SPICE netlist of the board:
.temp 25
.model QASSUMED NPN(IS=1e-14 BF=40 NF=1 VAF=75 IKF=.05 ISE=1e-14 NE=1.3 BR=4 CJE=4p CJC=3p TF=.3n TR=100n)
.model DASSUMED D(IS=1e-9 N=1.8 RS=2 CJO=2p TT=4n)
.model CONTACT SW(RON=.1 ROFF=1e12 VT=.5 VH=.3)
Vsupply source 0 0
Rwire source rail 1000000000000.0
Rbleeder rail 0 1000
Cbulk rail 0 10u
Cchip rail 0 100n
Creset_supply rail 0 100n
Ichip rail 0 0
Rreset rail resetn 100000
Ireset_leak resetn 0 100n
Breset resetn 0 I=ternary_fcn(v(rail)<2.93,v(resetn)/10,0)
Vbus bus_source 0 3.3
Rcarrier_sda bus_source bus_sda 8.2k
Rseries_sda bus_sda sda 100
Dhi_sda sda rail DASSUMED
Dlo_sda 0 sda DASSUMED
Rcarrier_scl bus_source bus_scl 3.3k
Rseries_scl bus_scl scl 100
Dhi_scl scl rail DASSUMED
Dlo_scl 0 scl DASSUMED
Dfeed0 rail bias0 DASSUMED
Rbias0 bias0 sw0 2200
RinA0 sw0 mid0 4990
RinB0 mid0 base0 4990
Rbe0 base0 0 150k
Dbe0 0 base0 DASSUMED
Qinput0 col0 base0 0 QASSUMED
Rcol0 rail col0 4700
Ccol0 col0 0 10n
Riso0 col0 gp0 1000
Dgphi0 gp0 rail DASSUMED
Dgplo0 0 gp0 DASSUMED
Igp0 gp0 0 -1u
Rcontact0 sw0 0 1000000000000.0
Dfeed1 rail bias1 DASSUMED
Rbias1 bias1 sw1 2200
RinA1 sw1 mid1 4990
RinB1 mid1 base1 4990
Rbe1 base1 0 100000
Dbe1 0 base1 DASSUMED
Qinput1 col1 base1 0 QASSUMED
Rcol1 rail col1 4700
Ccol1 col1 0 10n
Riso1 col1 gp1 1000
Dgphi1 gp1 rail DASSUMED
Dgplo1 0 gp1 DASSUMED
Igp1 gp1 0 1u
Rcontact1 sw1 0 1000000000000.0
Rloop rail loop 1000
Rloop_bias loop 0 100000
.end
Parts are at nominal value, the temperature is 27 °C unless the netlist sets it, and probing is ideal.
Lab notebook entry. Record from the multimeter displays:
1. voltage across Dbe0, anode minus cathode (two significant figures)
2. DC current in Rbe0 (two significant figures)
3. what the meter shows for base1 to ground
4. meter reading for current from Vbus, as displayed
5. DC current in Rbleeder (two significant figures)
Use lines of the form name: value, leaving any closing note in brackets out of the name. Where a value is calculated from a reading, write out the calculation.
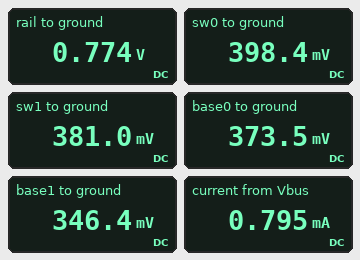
voltage across Dbe0, anode minus cathode: 0 V - 373.5 mV = -370 mV
DC current in Rbe0: (373.5 mV) / 150 kΩ = 2.5 µA
what the meter shows for base1 to ground: 346.4 mV
meter reading for current from Vbus, as displayed: 0.795 mA
DC current in Rbleeder: (774 mV) / 1 kΩ = 770 µA
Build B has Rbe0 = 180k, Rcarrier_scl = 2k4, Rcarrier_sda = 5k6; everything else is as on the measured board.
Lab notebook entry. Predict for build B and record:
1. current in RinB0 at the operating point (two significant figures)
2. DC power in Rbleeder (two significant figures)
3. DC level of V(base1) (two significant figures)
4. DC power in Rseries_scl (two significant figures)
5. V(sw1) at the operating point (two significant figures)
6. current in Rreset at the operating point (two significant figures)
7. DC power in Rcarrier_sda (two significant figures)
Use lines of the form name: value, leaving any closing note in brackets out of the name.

current in RinB0 at the operating point: 3.2 µA
DC power in Rbleeder: 910 µW
DC level of V(base1): 490 mV
DC power in Rseries_scl: 47 µW
V(sw1) at the operating point: 540 mV
current in Rreset at the operating point: 9.6 µA
DC power in Rcarrier_sda: 530 µW
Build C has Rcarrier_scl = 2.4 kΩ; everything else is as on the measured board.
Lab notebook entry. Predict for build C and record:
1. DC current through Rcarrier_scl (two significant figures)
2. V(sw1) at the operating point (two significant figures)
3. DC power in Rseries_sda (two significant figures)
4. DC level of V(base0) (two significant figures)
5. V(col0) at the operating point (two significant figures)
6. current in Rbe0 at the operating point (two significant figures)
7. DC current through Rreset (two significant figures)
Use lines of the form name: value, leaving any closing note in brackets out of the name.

DC current through Rcarrier_scl: 710 µA
V(sw1) at the operating point: 490 mV
DC power in Rseries_sda: 4.8 µW
DC level of V(base0): 480 mV
V(col0) at the operating point: 900 mV
current in Rbe0 at the operating point: 3.2 µA
DC current through Rreset: 9.0 µA
